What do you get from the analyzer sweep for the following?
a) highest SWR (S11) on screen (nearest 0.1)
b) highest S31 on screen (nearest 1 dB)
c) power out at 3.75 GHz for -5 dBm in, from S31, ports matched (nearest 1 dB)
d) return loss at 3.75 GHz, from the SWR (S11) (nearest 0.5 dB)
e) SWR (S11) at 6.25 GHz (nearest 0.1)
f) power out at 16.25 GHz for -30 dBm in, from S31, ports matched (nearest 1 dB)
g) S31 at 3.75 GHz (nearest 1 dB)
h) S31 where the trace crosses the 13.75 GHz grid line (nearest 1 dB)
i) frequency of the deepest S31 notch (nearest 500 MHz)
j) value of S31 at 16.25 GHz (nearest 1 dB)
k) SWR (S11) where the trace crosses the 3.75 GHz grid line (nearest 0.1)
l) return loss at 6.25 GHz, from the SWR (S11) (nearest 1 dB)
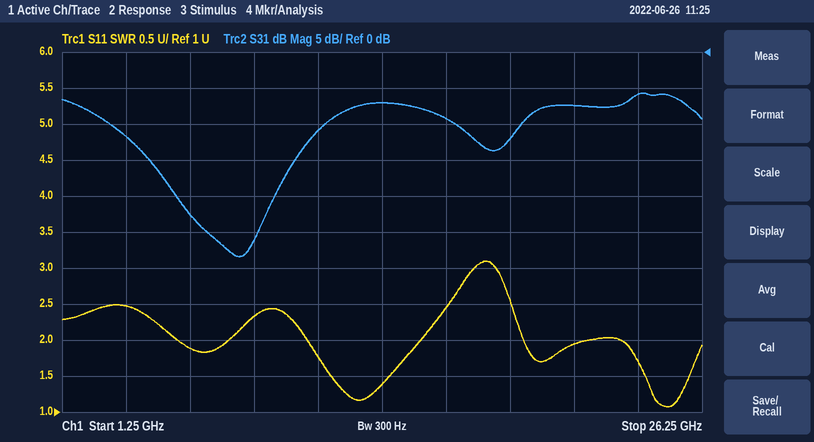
3.1
-6 dB
-17 dBm
7.5 dB
1.9
-39 dBm
-12 dB
-7 dB
8.0 GHz
-9 dB
2.5
10 dB
